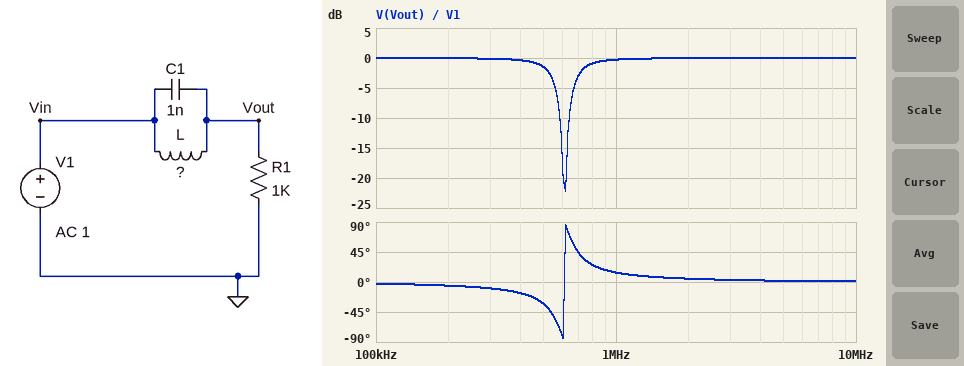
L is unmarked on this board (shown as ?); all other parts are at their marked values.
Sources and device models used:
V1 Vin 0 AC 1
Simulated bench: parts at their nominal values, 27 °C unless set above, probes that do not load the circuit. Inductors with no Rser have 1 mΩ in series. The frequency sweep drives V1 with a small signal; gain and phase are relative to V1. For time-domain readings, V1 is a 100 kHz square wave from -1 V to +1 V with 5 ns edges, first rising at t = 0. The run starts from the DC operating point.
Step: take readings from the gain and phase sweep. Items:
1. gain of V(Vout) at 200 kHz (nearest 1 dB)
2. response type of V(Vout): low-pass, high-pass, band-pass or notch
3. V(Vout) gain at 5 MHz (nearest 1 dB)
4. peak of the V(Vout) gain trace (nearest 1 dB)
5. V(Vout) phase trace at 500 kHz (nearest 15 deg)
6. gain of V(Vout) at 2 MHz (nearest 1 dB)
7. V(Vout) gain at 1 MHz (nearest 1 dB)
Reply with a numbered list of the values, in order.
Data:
1. 0 dB
2. notch
3. 0 dB
4. 0 dB
5. -30 deg
6. 0 dB
7. 0 dB
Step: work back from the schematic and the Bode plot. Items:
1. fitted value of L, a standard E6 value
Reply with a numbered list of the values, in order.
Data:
1. 68 µH
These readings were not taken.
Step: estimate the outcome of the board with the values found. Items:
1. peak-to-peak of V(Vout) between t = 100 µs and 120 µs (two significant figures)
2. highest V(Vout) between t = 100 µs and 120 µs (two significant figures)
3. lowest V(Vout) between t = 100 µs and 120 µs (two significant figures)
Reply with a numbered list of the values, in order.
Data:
1. 2.5 V
2. 1.3 V
3. -1.3 V
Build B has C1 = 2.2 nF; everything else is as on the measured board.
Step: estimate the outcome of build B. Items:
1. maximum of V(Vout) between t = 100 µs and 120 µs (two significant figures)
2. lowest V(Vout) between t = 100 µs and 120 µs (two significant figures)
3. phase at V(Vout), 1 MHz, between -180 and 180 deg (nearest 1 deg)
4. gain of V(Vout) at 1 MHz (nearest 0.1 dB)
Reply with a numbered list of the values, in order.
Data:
1. 1.2 V
2. -1.2 V
3. 5 deg
4. 0 dB
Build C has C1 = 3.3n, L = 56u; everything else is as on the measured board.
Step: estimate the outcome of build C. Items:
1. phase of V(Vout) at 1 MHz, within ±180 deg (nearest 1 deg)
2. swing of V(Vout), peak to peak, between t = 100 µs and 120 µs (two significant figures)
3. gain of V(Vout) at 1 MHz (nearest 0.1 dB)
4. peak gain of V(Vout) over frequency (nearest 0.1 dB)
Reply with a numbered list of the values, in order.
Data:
1. 3 deg
2. 2.3 V
3. 0 dB
4. 0 dB
